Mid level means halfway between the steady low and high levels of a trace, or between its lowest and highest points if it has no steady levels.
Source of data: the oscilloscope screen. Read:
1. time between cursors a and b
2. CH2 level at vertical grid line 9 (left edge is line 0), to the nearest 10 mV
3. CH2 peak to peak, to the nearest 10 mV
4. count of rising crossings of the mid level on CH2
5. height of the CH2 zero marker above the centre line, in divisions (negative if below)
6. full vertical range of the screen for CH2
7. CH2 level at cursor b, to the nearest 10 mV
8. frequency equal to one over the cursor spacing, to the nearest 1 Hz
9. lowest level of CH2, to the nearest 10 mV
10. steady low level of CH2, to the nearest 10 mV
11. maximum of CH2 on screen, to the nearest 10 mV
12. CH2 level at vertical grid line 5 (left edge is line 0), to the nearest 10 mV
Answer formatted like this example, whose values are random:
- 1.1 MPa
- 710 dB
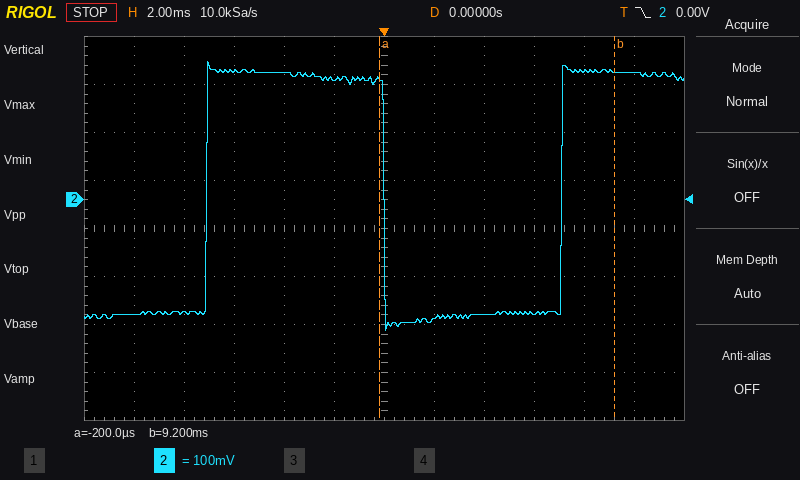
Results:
- 9.4 ms
- -240 mV
- 560 mV
- 2
- +0.6 div
- 800 mV
- 270 mV
- 106 Hz
- -270 mV
- -240 mV
- 290 mV
- 250 mV
